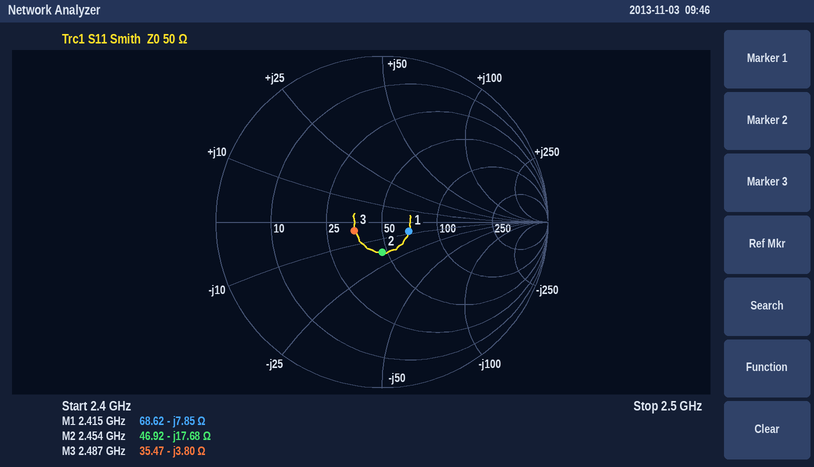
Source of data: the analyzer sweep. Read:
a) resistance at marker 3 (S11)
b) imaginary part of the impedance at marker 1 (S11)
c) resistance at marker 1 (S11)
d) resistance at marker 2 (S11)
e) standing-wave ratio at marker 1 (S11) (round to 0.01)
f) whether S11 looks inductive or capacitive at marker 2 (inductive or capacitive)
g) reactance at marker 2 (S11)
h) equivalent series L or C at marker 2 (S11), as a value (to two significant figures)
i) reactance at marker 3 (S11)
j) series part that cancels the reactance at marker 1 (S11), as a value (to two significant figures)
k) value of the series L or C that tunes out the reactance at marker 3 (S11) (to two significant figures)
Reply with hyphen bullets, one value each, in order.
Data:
- 35.47 Ω
- -7.85 Ω
- 68.62 Ω
- 46.92 Ω
- 1.41
- capacitive
- -17.68 Ω
- 3.7 pF
- -3.80 Ω
- 520 pH
- 240 pH
